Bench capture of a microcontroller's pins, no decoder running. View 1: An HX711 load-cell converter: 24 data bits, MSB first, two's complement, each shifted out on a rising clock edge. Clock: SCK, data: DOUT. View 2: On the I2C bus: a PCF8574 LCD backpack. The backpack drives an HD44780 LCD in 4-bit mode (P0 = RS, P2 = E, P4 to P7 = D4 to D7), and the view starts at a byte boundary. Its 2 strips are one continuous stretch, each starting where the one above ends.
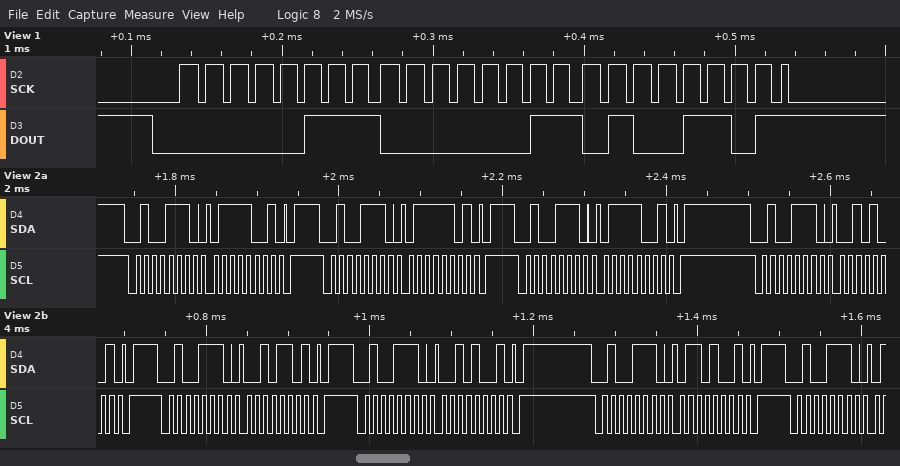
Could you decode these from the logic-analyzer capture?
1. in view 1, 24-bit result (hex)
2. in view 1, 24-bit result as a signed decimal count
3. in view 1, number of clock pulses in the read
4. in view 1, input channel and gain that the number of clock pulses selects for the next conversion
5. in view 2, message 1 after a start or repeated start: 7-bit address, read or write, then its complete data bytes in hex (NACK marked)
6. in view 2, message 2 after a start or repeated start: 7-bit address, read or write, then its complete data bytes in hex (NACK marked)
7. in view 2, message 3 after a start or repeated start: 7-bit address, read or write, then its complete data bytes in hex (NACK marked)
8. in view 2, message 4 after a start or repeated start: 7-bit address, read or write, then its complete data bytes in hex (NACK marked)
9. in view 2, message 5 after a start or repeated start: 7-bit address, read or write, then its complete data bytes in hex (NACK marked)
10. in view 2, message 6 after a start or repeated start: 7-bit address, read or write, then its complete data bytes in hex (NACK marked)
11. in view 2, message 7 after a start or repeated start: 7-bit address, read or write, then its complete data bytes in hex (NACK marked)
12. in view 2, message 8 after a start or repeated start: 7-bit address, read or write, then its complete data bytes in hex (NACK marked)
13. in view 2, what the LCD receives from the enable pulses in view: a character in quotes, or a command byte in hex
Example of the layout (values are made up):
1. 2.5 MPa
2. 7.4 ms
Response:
1. 0x07034D
2. 459597
3. 25
4. channel A, gain 128
5. 0x27 write: 79
6. 0x27 write: 7D
7. 0x27 write: 79
8. 0x27 write: 29
9. 0x27 write: 2D
10. 0x27 write: 29
11. 0x27 write: 69
12. 0x27 write
13. 'r'
